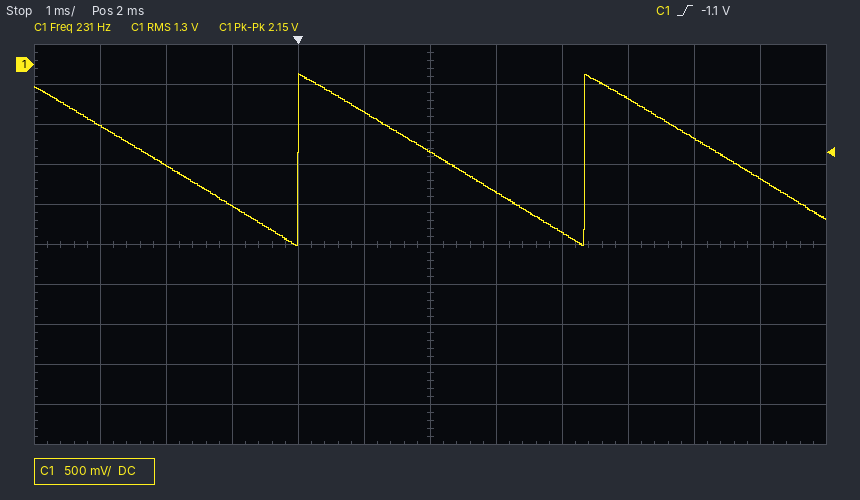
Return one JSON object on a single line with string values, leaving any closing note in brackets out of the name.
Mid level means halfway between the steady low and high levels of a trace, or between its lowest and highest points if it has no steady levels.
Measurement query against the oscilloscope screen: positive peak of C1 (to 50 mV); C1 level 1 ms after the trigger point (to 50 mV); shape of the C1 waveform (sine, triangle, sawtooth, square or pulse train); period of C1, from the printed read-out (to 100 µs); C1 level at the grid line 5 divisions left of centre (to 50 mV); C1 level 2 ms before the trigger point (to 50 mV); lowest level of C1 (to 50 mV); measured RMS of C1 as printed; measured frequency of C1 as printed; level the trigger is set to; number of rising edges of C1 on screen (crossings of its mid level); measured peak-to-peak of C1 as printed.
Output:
{"positive peak of C1": "-100 mV", "C1 level 1 ms after the trigger point": "-600 mV", "shape of the C1 waveform": "sawtooth", "period of C1, from the printed read-out": "4.3 ms", "C1 level at the grid line 5 divisions left of centre": "-750 mV", "C1 level 2 ms before the trigger point": "-1.25 V", "lowest level of C1": "-2.25 V", "measured RMS of C1 as printed": "1.3 V", "measured frequency of C1 as printed": "231 Hz", "level the trigger is set to": "-1.1 V", "number of rising edges of C1 on screen": "2", "measured peak-to-peak of C1 as printed": "2.15 V"}
